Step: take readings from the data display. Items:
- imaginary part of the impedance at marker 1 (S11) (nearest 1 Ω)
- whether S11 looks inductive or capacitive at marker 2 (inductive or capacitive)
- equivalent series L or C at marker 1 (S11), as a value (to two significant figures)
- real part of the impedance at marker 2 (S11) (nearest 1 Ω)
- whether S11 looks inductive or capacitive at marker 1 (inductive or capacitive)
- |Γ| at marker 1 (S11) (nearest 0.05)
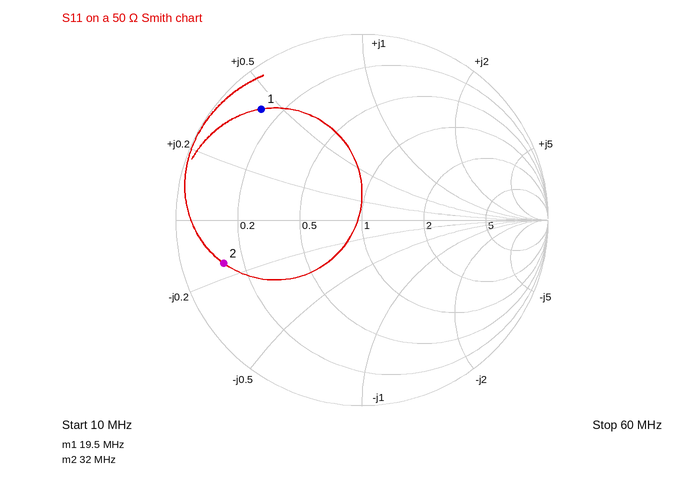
+22 Ω
capacitive
180 nH
6 Ω
inductive
0.80
